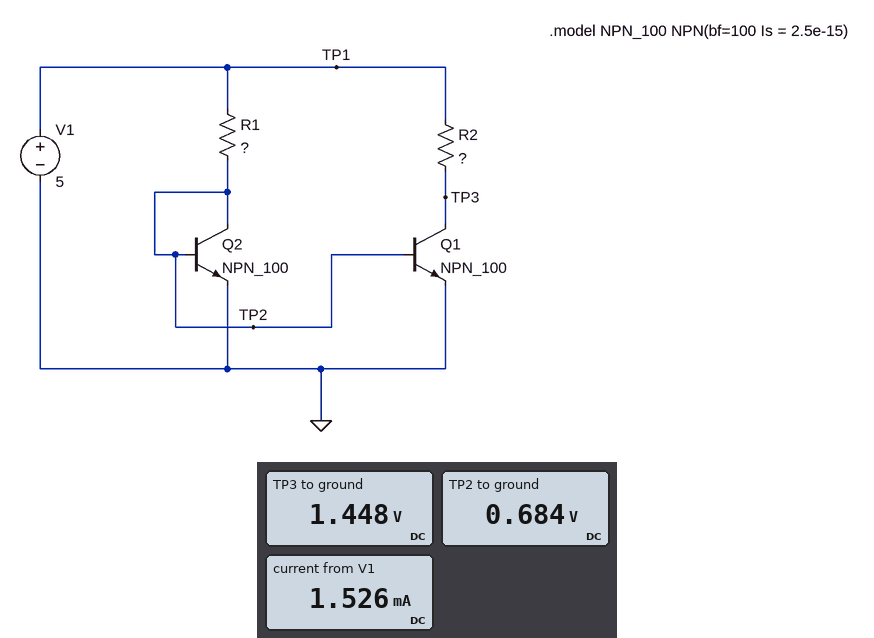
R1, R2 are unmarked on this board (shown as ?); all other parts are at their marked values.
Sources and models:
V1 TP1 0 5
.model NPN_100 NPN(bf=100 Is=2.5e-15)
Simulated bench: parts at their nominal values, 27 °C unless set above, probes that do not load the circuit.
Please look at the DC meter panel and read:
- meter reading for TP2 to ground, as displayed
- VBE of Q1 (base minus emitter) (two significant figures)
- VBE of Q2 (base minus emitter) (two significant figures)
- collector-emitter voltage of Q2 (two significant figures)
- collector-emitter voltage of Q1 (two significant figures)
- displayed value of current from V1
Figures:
0.684 V
680 mV
680 mV
680 mV
1.4 V
1.526 mA
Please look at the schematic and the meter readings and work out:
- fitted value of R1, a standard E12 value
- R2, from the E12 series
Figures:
5.6 kΩ
4.7 kΩ
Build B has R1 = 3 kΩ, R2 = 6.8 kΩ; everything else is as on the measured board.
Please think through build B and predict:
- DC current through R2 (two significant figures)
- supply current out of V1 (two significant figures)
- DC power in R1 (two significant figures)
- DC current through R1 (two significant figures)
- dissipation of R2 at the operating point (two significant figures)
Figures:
730 µA
2.2 mA
6.2 mW
1.4 mA
3.6 mW
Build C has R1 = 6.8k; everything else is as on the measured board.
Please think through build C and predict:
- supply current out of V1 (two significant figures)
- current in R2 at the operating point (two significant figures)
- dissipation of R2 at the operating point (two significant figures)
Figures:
1.3 mA
620 µA
1.8 mW
